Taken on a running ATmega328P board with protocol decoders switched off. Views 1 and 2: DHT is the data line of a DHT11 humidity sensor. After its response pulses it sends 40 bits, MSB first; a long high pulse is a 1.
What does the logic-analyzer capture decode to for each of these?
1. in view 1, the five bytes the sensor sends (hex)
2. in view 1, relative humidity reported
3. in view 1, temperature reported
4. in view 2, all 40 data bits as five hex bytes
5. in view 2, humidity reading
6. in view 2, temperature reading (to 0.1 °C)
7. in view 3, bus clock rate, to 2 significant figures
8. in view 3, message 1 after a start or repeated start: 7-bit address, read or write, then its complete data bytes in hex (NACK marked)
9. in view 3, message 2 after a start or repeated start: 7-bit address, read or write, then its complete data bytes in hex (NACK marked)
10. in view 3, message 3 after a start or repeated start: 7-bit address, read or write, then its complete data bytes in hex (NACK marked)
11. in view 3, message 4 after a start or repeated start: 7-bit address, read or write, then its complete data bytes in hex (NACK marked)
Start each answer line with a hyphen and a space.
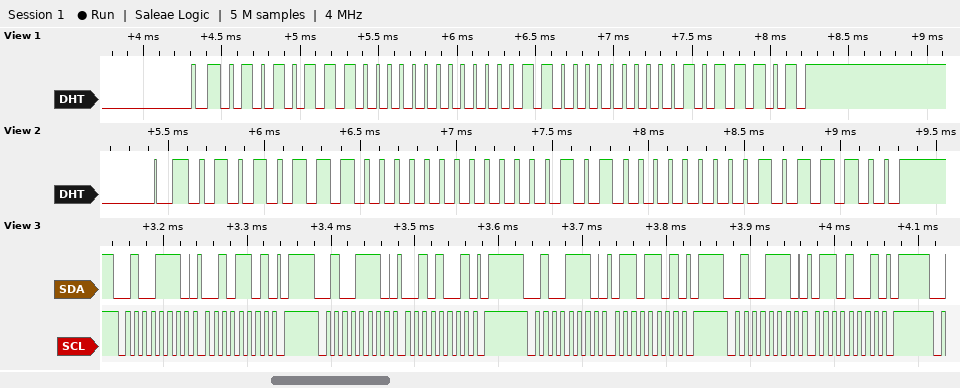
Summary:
- 57 00 06 00 5D
- 87 %
- 6.0 °C
- 57 00 05 00 5C
- 87 %
- 5.0 °C
- 100 kHz
- 0x27 write: 2D
- 0x27 write: 29
- 0x27 write: 6D
- 0x27 write: 69
